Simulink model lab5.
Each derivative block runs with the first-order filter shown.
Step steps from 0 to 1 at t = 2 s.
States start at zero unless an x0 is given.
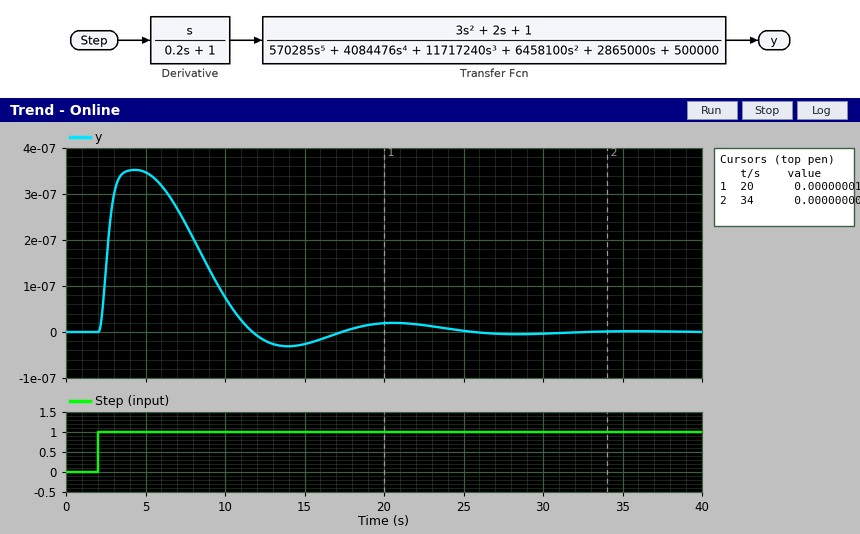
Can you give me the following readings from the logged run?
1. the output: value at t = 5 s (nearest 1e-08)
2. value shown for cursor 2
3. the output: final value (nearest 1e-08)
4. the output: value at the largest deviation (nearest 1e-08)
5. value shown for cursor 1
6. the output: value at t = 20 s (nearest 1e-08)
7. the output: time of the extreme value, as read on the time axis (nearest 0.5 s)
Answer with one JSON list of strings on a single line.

["0.00000035", "0.000000001", "0.00000000", "0.00000035", "0.000000019", "0.00000002", "4.5 s"]
